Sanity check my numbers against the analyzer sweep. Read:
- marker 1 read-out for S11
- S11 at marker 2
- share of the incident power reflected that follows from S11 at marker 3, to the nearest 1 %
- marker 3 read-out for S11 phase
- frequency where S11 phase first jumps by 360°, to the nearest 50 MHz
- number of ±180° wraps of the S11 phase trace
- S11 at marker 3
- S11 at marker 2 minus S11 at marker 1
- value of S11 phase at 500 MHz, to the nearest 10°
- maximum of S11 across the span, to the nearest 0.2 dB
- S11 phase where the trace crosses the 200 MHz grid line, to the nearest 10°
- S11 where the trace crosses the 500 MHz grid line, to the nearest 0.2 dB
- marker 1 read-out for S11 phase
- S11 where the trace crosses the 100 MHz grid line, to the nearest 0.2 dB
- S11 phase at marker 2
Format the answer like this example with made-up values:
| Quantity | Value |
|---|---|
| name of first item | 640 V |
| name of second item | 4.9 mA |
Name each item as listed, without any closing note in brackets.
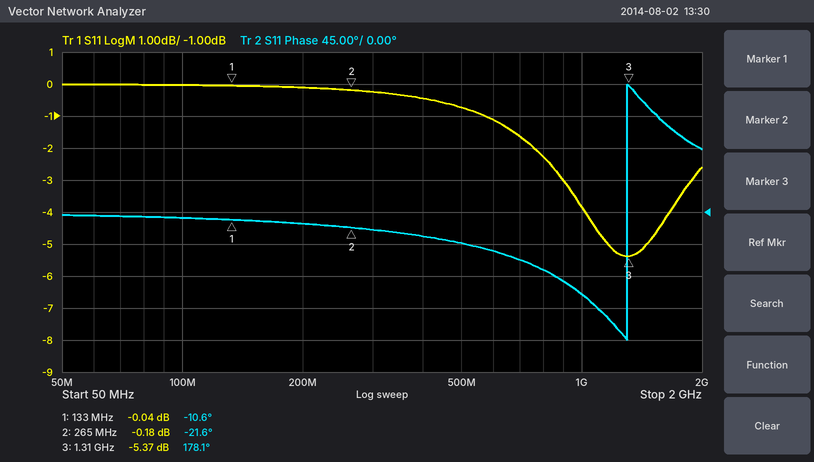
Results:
| Quantity | Value |
|---|---|
| marker 1 read-out for S11 | -0.04 dB |
| S11 at marker 2 | -0.18 dB |
| share of the incident power reflected that follows from S11 at marker 3, to the nearest 1 % | 29 % |
| marker 3 read-out for S11 phase | 178.1° |
| frequency where S11 phase first jumps by 360°, to the nearest 50 MHz | 1.30 GHz |
| number of ±180° wraps of the S11 phase trace | 1 |
| S11 at marker 3 | -5.37 dB |
| S11 at marker 2 minus S11 at marker 1 | -0.14 dB |
| value of S11 phase at 500 MHz, to the nearest 10° | -40° |
| maximum of S11 across the span, to the nearest 0.2 dB | 0.0 dB |
| S11 phase where the trace crosses the 200 MHz grid line, to the nearest 10° | -20° |
| S11 where the trace crosses the 500 MHz grid line, to the nearest 0.2 dB | -0.8 dB |
| marker 1 read-out for S11 phase | -10.6° |
| S11 where the trace crosses the 100 MHz grid line, to the nearest 0.2 dB | 0.0 dB |
| S11 phase at marker 2 | -21.6° |
